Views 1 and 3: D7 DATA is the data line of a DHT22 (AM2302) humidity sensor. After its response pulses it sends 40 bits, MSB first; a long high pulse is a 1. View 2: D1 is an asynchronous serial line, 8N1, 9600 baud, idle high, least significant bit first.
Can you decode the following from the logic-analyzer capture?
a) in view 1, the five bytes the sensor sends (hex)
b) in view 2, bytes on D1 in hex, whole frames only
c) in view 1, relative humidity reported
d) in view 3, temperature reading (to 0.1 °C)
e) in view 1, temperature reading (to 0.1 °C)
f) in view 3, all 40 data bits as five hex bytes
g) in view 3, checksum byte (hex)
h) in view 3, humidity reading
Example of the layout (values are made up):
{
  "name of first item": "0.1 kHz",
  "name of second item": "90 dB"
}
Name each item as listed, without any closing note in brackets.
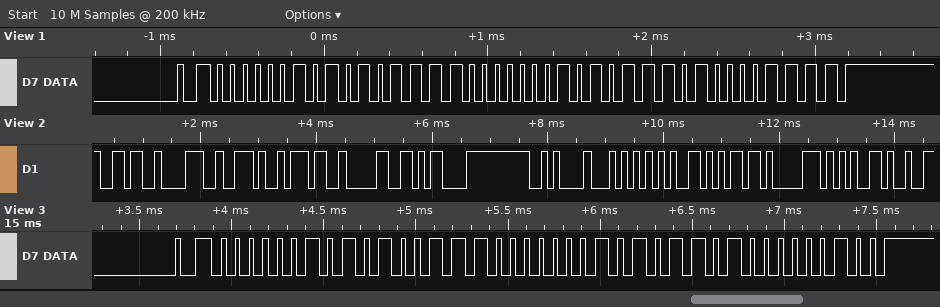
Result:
{
  "in view 1, the five bytes the sensor sends": "02 AF 01 5D 0F",
  "in view 2, bytes on D1 in hex, whole frames only": "36 38 2E 37 30 0D 0A 54 65 6D 70 65",
  "in view 1, relative humidity reported": "68.7 %",
  "in view 3, temperature reading": "34.6 °C",
  "in view 1, temperature reading": "34.9 °C",
  "in view 3, all 40 data bits as five hex bytes": "02 A7 01 5A 04",
  "in view 3, checksum byte": "0x04",
  "in view 3, humidity reading": "67.9 %"
}
